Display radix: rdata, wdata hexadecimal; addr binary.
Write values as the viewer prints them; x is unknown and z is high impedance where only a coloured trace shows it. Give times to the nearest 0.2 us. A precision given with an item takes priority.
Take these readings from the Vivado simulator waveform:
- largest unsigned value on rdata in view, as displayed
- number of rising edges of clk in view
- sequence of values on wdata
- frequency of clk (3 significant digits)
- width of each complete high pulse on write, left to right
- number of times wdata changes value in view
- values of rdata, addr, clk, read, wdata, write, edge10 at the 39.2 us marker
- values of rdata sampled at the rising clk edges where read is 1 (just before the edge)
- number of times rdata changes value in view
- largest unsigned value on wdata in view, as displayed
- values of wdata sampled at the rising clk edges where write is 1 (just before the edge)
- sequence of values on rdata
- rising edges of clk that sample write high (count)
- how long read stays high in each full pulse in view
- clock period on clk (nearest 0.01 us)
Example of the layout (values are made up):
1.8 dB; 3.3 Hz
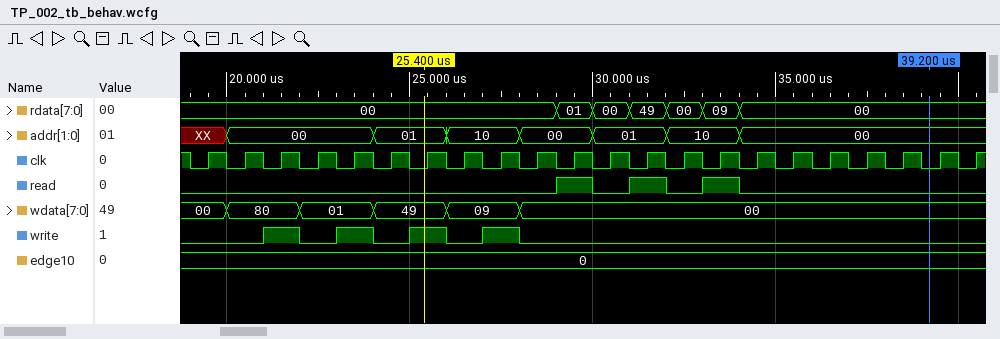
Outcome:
49; 22; 00, 80, 01, 49, 09, 00; 1.00 MHz; 1 us, 1 us, 1 us, 1 us; 5; rdata=00, addr=00, clk=0, read=0, wdata=00, write=0, edge10=0; 01, 49, 09; 6; 80; 80, 01, 49, 09; 00, 01, 00, 49, 00, 09, 00; 4; 1 us, 1 us, 1 us; 1 us
